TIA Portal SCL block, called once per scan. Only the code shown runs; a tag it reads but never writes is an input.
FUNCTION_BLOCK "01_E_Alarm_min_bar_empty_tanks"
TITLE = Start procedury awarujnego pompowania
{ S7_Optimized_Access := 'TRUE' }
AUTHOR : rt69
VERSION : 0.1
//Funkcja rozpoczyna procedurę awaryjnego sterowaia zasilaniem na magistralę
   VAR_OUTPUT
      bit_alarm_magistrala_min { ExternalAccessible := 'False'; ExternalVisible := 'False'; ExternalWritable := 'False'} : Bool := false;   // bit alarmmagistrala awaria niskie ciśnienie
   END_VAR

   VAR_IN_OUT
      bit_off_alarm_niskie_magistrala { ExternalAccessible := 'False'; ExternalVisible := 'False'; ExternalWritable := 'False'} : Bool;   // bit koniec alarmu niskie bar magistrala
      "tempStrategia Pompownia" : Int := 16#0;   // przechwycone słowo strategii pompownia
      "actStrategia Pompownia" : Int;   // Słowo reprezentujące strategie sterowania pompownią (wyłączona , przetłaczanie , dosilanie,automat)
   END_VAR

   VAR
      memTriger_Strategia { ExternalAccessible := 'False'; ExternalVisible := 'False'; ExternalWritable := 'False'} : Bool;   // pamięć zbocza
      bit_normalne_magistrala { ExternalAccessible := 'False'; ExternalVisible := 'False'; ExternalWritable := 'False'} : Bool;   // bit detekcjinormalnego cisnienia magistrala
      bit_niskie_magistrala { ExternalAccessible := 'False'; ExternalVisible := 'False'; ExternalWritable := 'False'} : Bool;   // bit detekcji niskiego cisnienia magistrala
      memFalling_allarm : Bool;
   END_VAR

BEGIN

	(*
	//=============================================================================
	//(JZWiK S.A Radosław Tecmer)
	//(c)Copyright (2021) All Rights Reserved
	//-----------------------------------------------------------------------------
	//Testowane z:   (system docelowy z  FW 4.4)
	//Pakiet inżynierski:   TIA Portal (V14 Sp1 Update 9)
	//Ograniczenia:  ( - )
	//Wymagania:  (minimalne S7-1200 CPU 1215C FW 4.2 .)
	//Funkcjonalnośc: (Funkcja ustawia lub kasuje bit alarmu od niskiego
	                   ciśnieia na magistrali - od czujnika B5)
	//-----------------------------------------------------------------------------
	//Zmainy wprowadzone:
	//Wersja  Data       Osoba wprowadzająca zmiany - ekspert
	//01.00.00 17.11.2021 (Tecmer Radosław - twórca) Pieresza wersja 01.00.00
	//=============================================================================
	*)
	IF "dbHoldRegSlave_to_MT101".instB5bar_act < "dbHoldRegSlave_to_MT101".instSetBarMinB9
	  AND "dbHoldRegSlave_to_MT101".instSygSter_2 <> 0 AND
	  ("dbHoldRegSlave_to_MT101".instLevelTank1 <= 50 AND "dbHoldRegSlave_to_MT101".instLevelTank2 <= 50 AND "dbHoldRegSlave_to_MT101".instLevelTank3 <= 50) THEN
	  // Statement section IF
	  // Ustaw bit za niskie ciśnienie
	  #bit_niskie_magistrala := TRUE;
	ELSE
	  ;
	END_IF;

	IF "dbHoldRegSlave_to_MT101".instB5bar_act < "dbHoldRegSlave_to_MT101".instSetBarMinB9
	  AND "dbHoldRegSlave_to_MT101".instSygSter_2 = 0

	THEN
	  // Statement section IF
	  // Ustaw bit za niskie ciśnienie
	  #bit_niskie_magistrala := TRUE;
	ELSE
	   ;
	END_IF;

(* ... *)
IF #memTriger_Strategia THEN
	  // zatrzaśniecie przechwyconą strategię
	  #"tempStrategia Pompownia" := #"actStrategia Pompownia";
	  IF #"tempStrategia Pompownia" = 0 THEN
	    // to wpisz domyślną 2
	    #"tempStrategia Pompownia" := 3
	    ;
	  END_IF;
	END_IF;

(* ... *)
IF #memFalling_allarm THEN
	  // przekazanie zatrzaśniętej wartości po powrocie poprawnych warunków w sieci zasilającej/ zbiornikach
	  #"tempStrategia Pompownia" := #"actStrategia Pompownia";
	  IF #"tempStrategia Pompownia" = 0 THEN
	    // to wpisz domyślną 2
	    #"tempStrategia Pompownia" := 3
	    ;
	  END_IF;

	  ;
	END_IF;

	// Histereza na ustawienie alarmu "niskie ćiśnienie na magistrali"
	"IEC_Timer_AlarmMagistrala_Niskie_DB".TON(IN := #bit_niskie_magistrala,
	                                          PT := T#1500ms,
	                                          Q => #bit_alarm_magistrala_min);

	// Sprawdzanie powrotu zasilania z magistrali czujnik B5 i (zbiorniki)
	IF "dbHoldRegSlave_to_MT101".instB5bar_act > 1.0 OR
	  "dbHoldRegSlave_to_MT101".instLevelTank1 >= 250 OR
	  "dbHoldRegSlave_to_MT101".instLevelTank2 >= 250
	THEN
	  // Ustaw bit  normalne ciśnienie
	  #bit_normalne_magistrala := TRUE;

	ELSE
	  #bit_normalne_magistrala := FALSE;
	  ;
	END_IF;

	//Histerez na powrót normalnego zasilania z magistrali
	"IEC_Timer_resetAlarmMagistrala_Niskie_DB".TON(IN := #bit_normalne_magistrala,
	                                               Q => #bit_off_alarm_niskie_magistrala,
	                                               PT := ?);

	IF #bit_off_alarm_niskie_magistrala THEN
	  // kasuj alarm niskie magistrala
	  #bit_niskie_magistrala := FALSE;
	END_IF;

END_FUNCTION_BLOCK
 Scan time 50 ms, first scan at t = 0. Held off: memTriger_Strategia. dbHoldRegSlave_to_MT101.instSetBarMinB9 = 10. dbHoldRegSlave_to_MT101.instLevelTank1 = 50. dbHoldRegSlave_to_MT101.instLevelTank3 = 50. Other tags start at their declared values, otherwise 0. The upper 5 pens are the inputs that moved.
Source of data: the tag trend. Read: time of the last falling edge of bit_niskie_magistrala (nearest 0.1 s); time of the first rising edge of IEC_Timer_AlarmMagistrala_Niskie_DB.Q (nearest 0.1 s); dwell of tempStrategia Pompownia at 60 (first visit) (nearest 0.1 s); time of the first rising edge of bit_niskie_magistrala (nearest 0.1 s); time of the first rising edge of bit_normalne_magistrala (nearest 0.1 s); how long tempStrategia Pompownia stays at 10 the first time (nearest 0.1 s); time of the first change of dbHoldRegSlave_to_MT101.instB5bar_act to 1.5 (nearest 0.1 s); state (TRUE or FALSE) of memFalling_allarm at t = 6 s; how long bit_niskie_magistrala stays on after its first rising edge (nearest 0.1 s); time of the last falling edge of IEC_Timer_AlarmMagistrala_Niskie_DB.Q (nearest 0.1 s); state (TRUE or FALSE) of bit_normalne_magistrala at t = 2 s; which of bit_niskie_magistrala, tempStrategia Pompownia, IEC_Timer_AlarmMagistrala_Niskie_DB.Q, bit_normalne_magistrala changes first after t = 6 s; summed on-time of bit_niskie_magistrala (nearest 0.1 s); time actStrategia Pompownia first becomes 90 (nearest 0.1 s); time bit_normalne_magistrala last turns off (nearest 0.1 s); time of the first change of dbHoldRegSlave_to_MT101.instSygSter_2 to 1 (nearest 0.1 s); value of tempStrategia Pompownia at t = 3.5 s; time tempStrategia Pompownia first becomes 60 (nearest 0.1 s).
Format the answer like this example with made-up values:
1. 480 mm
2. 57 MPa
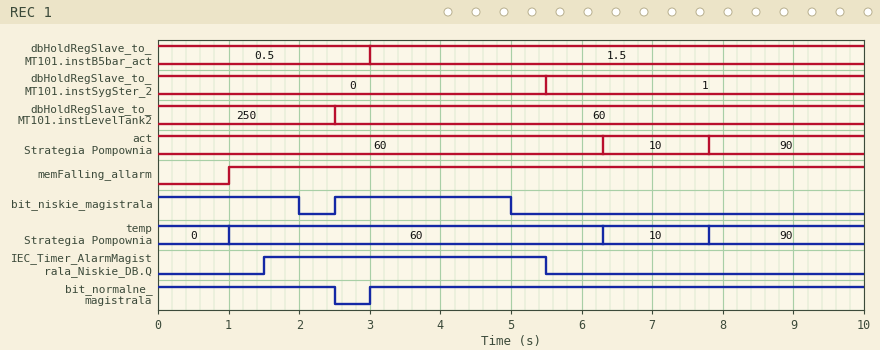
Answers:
1. 5.0 s
2. 1.5 s
3. 5.3 s
4. 2.5 s
5. 3.0 s
6. 1.5 s
7. 3.0 s
8. TRUE
9. 2.5 s
10. 5.5 s
11. TRUE
12. tempStrategia Pompownia
13. 4.5 s
14. 7.8 s
15. 2.5 s
16. 5.5 s
17. 60
18. 1.0 s
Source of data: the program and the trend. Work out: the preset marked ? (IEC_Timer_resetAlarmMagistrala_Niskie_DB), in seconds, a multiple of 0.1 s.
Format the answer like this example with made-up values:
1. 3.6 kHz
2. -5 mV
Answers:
1. 2.0 s
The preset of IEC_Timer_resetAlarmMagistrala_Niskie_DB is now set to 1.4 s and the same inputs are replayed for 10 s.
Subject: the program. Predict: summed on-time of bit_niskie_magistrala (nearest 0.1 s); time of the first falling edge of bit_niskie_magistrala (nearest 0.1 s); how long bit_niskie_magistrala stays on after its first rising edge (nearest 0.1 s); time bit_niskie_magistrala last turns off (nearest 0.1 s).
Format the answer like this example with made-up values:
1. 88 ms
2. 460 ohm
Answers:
1. 3.3 s
2. 1.4 s
3. 1.9 s
4. 4.4 s
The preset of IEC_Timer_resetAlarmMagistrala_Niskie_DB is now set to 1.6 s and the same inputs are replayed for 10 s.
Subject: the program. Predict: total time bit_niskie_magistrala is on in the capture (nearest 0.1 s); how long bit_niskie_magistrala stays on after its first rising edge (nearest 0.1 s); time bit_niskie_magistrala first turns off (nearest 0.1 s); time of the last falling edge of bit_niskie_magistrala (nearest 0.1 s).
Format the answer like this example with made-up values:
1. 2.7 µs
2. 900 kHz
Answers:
1. 3.7 s
2. 2.1 s
3. 1.6 s
4. 4.6 s
